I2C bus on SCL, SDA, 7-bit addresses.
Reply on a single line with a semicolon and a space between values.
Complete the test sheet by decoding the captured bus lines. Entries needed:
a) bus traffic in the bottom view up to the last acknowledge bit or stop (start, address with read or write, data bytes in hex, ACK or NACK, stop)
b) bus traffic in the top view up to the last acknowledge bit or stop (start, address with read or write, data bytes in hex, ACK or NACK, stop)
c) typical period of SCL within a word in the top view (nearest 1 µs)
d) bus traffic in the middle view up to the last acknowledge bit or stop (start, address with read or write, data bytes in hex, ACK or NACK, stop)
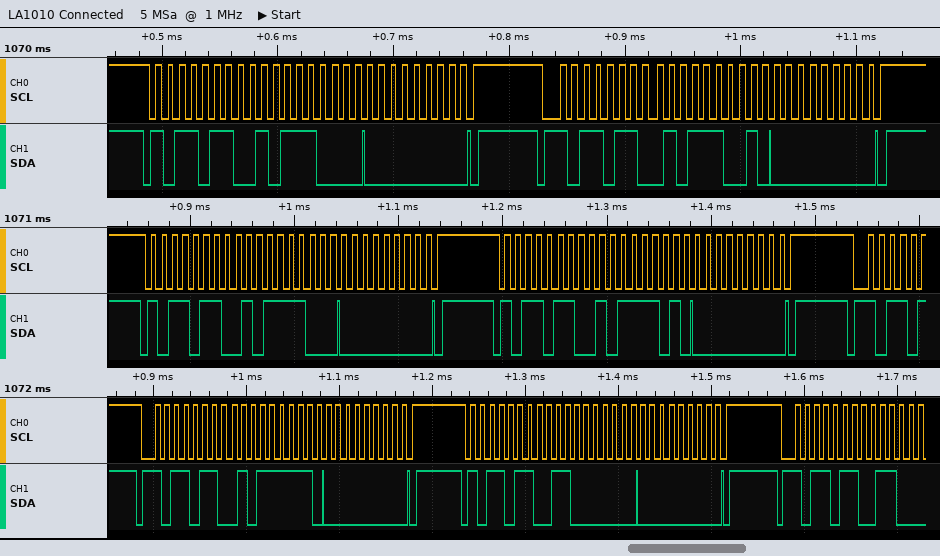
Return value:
start, address 5B write ACK, BF ACK, 00 ACK, stop, start, address 5B write ACK, C0 ACK, 00 ACK, stop, start, address 5B write ACK; start, address 5B write ACK, B8 ACK, 00 ACK, stop, start, address 5B write ACK, B9 ACK, 00 ACK, stop; 10 µs; start, address 5B write ACK, BC ACK, 00 ACK, stop, start, address 5B write ACK, BD ACK, 00 ACK, stop
